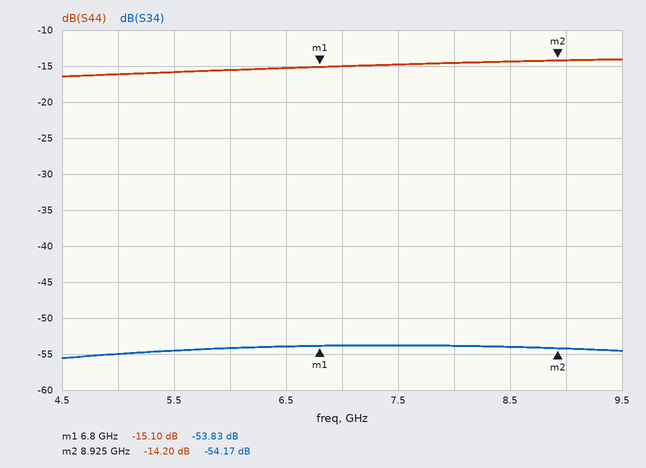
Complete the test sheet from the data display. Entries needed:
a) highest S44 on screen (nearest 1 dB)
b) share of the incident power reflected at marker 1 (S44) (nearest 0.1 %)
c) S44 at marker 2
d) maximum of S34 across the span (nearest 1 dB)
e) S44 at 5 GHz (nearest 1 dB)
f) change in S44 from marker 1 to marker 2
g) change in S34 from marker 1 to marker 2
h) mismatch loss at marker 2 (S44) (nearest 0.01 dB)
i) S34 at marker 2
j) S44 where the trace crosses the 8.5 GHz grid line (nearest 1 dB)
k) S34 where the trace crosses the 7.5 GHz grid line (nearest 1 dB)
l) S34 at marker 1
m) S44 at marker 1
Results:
-14 dB
3.1 %
-14.20 dB
-54 dB
-16 dB
0.90 dB
-0.34 dB
0.17 dB
-54.17 dB
-14 dB
-54 dB
-53.83 dB
-15.10 dB
